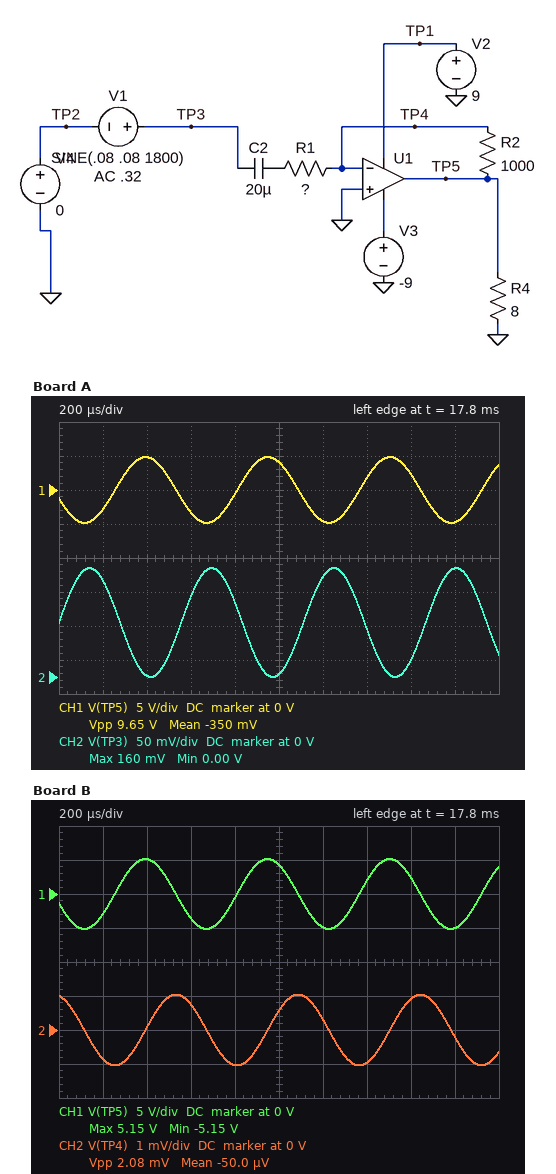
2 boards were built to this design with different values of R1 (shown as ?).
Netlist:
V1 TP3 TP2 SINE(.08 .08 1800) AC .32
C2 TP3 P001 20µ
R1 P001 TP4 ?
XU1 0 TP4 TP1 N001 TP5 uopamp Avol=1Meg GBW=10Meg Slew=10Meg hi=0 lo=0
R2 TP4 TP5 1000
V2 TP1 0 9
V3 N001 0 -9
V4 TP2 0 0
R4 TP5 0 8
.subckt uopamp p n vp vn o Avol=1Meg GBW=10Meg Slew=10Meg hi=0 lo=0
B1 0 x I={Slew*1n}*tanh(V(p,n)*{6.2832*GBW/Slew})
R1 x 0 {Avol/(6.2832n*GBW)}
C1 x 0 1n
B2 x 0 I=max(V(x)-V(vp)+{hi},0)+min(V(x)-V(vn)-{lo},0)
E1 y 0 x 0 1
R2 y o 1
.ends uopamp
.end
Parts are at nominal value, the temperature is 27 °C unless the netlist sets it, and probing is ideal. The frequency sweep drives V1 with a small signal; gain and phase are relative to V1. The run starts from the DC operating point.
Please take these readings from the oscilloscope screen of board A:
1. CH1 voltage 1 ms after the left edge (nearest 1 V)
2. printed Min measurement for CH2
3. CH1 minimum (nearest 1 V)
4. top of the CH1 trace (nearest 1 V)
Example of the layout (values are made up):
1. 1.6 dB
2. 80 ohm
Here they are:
1. 4 V
2. 0.00 V
3. -5 V
4. 5 V
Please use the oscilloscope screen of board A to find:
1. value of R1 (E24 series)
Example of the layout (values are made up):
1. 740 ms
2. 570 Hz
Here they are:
1. 16 Ω
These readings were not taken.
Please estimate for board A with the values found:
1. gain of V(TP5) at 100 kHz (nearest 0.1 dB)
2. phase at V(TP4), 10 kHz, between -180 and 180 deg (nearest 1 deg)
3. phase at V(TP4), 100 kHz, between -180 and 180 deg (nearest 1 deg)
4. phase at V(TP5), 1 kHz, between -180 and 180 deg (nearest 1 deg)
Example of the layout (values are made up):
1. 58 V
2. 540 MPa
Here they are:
1. 34.1 dB
2. 89 deg
3. 55 deg
4. -154 deg
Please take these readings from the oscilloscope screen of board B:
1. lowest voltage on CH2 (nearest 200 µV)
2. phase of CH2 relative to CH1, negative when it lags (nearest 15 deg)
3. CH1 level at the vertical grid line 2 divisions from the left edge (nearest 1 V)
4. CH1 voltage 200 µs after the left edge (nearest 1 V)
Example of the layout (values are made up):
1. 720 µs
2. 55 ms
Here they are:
1. -1.0 mV
2. -90 deg
3. 5 V
4. -3 V
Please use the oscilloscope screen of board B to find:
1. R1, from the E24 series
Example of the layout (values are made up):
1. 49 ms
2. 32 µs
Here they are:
1. 15 Ω
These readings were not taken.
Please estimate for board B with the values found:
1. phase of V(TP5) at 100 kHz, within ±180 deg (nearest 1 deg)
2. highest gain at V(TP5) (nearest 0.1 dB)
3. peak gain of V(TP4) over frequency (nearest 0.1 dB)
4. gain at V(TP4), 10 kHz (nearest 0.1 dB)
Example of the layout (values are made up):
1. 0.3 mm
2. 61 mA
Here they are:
1. 143 deg
2. 36.5 dB
3. -0.1 dB
4. -22.5 dB
